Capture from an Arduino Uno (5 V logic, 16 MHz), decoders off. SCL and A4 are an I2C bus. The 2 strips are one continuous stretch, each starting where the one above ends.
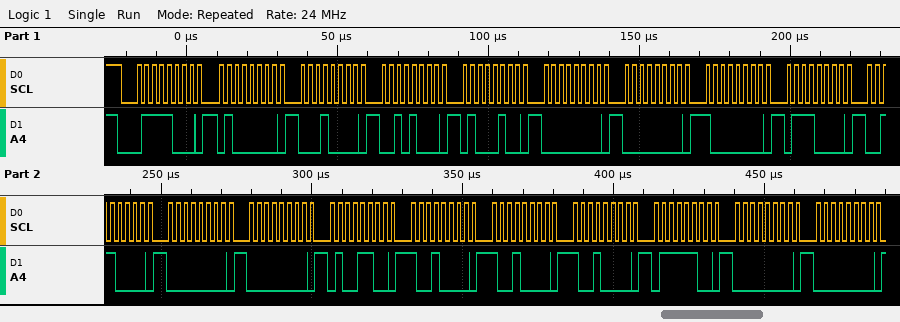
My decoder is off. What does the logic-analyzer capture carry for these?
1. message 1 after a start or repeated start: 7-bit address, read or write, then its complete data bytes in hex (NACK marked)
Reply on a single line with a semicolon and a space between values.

0x3C write: 40 10 28 44 00 00 80 70 30 00 00 4C 90 90 90 7C 00 00
